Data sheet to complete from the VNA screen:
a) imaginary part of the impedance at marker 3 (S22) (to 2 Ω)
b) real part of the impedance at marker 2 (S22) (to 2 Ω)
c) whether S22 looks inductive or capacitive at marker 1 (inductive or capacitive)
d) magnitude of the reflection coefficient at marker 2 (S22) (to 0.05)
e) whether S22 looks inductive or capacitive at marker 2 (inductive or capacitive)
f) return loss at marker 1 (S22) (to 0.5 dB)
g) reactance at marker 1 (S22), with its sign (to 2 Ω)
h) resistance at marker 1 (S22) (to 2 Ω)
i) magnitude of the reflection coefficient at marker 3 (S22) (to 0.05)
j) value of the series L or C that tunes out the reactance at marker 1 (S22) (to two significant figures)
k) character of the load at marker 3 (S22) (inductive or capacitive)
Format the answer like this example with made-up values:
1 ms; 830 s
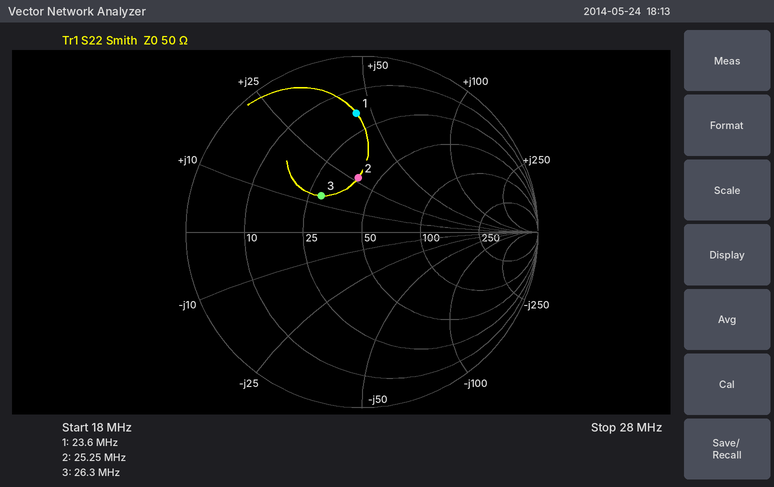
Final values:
+14 Ω; 40 Ω; inductive; 0.30; inductive; 3.5 dB; +44 Ω; 18 Ω; 0.30; 150 pF; inductive
